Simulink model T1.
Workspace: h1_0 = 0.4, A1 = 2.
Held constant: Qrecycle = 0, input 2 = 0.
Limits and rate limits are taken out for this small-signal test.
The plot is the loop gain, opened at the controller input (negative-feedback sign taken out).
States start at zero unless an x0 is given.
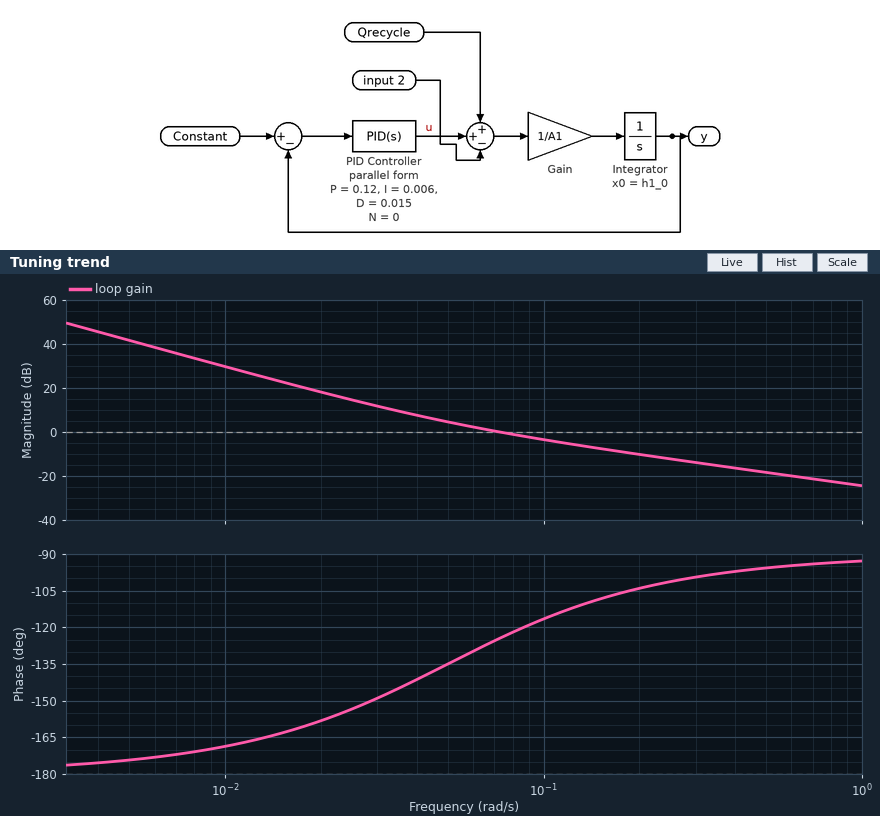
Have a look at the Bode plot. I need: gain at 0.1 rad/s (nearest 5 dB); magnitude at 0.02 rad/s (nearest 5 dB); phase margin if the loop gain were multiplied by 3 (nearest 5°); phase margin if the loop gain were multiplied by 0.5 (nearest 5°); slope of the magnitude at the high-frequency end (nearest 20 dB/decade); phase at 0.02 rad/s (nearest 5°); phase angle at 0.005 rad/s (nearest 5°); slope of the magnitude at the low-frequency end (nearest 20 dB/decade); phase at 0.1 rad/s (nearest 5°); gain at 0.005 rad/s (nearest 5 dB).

-5 dB
20 dB
75°
40°
-20 dB/decade
-160°
-175°
-40 dB/decade
-115°
40 dB
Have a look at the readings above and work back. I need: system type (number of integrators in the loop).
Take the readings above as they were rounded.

2
